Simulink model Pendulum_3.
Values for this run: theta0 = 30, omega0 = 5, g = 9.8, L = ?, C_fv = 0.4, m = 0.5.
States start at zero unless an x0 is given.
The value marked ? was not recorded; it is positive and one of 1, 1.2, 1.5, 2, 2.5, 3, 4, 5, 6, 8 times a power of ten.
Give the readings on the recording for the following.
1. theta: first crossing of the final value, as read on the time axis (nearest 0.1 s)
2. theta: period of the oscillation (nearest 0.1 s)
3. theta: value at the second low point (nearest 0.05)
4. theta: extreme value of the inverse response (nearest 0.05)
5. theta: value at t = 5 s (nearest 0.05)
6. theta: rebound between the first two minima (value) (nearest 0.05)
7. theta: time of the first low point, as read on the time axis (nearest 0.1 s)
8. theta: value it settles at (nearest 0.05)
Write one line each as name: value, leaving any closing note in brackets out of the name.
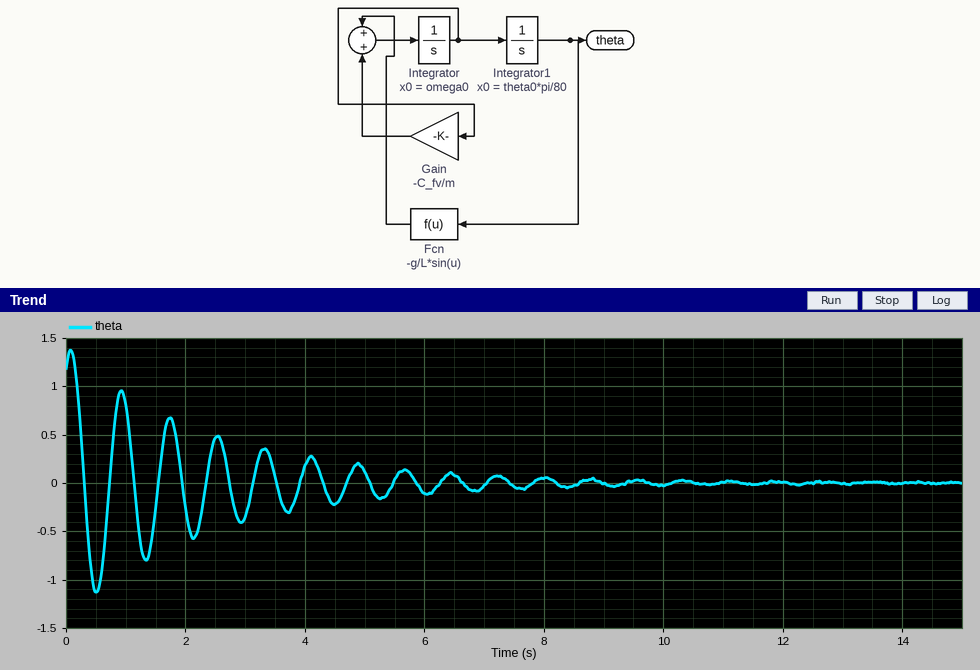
theta: first crossing of the final value, as read on the time axis: 0.3 s
theta: period of the oscillation: 0.8 s
theta: value at the second low point: -0.80
theta: extreme value of the inverse response: 1.35
theta: value at t = 5 s: 0.10
theta: rebound between the first two minima (value): 0.95
theta: time of the first low point, as read on the time axis: 0.5 s
theta: value it settles at: 0.00
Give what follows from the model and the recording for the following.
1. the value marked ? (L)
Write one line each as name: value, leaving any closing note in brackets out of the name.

the value marked ?: 0.15
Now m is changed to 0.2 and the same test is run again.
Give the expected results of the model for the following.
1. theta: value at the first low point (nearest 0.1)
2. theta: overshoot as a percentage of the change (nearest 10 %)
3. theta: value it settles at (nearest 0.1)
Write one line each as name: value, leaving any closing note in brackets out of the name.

theta: value at the first low point: -0.9
theta: overshoot as a percentage of the change: 70 %
theta: value it settles at: 0.0
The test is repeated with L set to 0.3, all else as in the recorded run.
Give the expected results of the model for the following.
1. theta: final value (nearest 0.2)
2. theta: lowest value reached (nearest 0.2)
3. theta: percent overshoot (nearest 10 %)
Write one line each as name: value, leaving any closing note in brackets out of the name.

theta: final value: 0.0
theta: lowest value reached: -1.2
theta: percent overshoot: 100 %
